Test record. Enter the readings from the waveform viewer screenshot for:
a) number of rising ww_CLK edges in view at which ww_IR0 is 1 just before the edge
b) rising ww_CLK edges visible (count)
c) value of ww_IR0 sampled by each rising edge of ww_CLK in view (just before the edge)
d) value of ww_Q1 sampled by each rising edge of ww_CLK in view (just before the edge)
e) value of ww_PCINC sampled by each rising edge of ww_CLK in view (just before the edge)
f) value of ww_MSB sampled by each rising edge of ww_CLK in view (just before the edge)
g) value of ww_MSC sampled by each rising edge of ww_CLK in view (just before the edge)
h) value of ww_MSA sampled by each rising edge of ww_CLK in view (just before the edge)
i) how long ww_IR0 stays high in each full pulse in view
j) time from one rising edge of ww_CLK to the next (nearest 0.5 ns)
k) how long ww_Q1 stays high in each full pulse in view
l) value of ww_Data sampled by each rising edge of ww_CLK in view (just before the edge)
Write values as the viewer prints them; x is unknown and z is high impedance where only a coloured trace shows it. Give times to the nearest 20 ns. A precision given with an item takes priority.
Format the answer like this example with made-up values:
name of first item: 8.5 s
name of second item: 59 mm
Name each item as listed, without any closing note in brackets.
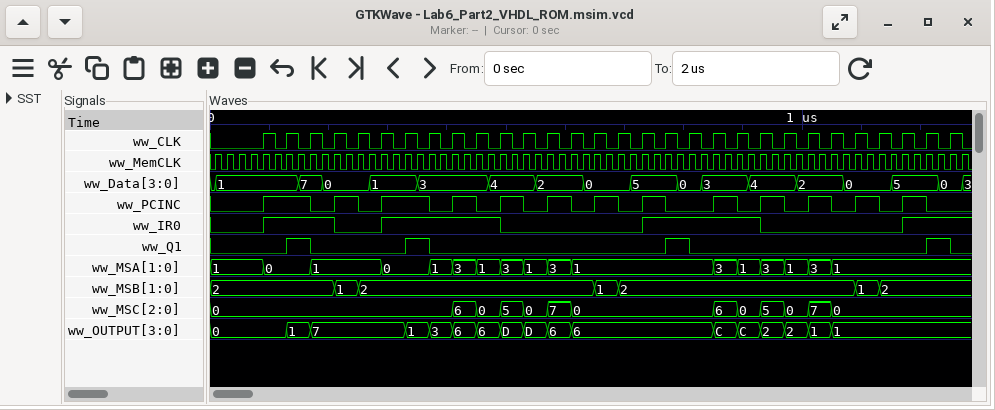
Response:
number of rising ww_CLK edges in view at which ww_IR0 is 1 just before the edge: 15
rising ww_CLK edges visible: 30
value of ww_IR0 sampled by each rising edge of ww_CLK in view: 0 1 1 1 0 0 1 1 1 1 1 0 0 0 0 0 0 1 1 1 1 1 0 0 0 0 0 0 1 1
value of ww_Q1 sampled by each rising edge of ww_CLK in view: 0 0 1 0 0 0 0 1 0 0 0 0 0 0 0 0 0 0 1 0 0 0 0 0 0 0 0 0 0 1
value of ww_PCINC sampled by each rising edge of ww_CLK in view: 0 1 1 0 1 0 1 1 0 1 0 1 0 1 0 1 0 1 0 0 1 0 1 0 1 0 1 0 1 0
value of ww_MSB sampled by each rising edge of ww_CLK in view: 2, 2, 2, 2, 1, 2, 2, 2, 2, 2, 2, 2, 2, 2, 2, 1, 2, 2, 2, 2, 2, 2, 2, 2, 2, 2, 1, 2, 2, 2
value of ww_MSC sampled by each rising edge of ww_CLK in view: 0, 0, 0, 0, 0, 0, 0, 0, 0, 6, 0, 5, 0, 7, 0, 0, 0, 0, 0, 0, 6, 0, 5, 0, 7, 0, 0, 0, 0, 0
value of ww_MSA sampled by each rising edge of ww_CLK in view: 1, 0, 0, 1, 1, 1, 0, 0, 1, 3, 1, 3, 1, 3, 1, 1, 1, 1, 1, 1, 3, 1, 3, 1, 3, 1, 1, 1, 1, 1
how long ww_IR0 stays high in each full pulse in view: 120 ns, 200 ns, 200 ns
time from one rising edge of ww_CLK to the next: 40 ns
how long ww_Q1 stays high in each full pulse in view: 40 ns, 40 ns, 40 ns, 40 ns
value of ww_Data sampled by each rising edge of ww_CLK in view: 1, 1, 7, 0, 0, 1, 1, 3, 3, 3, 4, 4, 2, 2, 0, 0, 5, 5, 0, 3, 3, 4, 4, 2, 2, 0, 0, 5, 5, 0
